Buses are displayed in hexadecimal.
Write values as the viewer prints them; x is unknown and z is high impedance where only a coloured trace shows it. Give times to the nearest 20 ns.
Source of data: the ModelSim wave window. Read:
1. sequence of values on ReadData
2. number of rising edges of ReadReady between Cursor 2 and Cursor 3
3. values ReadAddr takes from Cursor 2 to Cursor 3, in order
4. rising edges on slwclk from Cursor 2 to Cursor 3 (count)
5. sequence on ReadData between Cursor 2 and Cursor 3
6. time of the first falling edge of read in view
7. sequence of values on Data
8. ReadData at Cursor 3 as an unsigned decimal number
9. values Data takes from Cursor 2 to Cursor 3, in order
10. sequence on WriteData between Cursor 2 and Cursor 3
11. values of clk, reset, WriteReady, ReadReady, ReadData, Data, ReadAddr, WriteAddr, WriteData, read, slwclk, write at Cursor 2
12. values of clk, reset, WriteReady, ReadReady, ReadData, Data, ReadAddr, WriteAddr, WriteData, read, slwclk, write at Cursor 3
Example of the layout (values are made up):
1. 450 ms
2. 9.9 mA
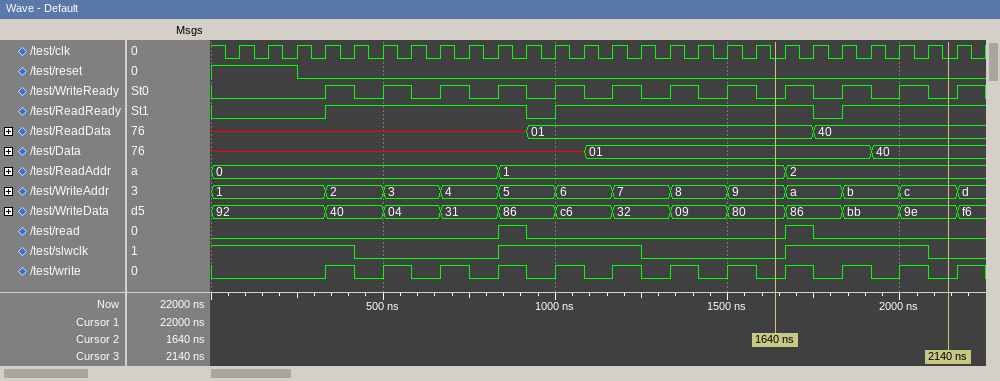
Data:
1. x, 01, 40
2. 1
3. 1, 2
4. 1
5. 01, 40
6. 920 ns
7. x, 01, 40
8. 64
9. 01, 40
10. 80, 86, bb, 9e
11. clk=0, reset=0, WriteReady=0, ReadReady=1, ReadData=01, Data=01, ReadAddr=1, WriteAddr=9, WriteData=80, read=0, slwclk=0, write=0
12. clk=0, reset=0, WriteReady=0, ReadReady=1, ReadData=40, Data=40, ReadAddr=2, WriteAddr=c, WriteData=9e, read=0, slwclk=0, write=0
